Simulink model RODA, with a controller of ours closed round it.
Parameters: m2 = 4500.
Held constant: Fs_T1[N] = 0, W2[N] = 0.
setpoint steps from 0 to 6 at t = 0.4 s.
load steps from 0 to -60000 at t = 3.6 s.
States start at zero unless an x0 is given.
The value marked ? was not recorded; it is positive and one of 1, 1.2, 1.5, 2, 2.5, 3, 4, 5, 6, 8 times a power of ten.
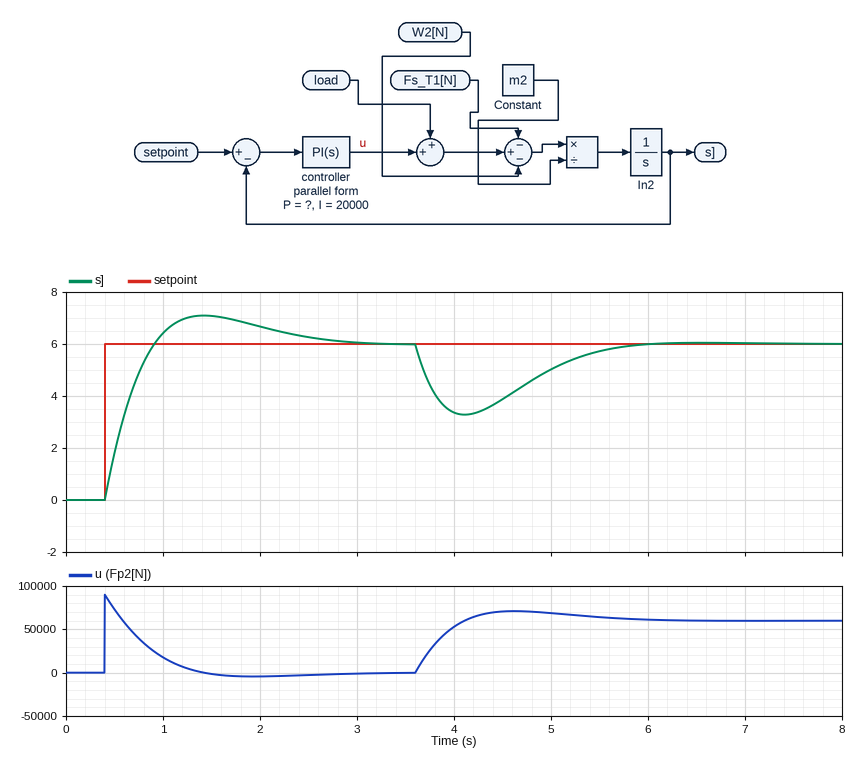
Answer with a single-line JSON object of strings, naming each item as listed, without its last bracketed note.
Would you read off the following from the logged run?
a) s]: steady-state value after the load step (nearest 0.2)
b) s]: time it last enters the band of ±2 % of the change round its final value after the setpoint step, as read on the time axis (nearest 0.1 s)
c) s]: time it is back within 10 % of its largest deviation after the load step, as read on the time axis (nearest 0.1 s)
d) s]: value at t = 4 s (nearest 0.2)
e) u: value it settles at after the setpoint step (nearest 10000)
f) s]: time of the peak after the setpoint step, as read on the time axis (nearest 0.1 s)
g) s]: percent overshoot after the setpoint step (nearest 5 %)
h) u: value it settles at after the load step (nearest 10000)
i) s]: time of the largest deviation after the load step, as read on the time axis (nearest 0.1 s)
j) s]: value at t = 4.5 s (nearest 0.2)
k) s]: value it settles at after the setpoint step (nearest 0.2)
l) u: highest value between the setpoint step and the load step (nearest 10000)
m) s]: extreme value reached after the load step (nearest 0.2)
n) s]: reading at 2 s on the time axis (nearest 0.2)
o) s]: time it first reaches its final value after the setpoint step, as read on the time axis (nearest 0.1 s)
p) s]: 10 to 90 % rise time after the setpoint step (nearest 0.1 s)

{"s]: steady-state value after the load step": "6.0", "s]: time it last enters the band of ±2 % of the change round its final value after the setpoint step, as read on the time axis": "2.8 s", "s]: time it is back within 10 % of its largest deviation after the load step, as read on the time axis": "5.5 s", "s]: value at t = 4 s": "3.4", "u: value it settles at after the setpoint step": "0", "s]: time of the peak after the setpoint step, as read on the time axis": "1.4 s", "s]: percent overshoot after the setpoint step": "20 %", "u: value it settles at after the load step": "60000", "s]: time of the largest deviation after the load step, as read on the time axis": "4.1 s", "s]: value at t = 4.5 s": "3.8", "s]: value it settles at after the setpoint step": "6.0", "u: highest value between the setpoint step and the load step": "90000", "s]: extreme value reached after the load step": "3.2", "s]: reading at 2 s on the time axis": "6.6", "s]: time it first reaches its final value after the setpoint step, as read on the time axis": "0.9 s", "s]: 10 to 90 % rise time after the setpoint step": "0.4 s"}
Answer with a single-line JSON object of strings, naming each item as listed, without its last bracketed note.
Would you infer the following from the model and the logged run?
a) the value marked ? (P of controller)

{"the value marked ?": "15000"}
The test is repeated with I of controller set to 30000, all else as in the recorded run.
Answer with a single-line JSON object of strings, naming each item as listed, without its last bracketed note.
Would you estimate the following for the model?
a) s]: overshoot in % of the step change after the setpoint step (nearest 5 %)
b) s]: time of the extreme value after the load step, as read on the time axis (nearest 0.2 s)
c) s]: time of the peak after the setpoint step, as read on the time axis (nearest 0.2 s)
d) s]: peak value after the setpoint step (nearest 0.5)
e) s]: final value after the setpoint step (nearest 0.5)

{"s]: overshoot in % of the step change after the setpoint step": "25 %", "s]: time of the extreme value after the load step, as read on the time axis": "4.0 s", "s]: time of the peak after the setpoint step, as read on the time axis": "1.2 s", "s]: peak value after the setpoint step": "7.5", "s]: final value after the setpoint step": "6.0"}
